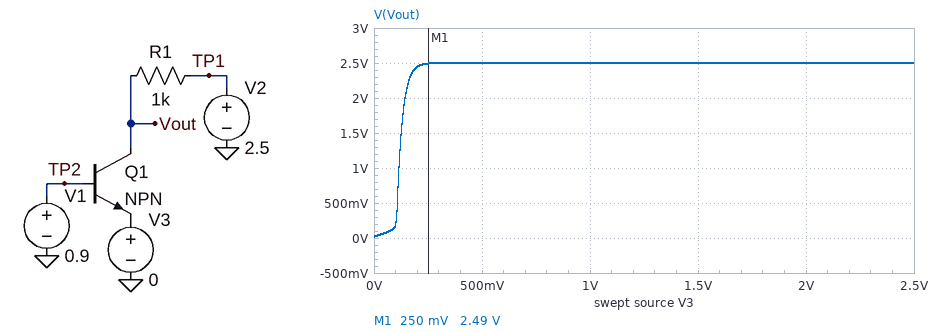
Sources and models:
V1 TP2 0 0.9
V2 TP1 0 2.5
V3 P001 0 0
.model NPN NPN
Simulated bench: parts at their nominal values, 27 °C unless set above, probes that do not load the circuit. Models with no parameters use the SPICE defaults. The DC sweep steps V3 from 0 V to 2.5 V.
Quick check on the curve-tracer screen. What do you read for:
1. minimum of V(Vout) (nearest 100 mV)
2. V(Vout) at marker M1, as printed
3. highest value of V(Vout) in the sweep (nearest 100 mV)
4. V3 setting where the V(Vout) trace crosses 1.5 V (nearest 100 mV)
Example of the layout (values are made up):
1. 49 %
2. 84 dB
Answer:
1. 0 V
2. 2.49 V
3. 2.5 V
4. 100 mV
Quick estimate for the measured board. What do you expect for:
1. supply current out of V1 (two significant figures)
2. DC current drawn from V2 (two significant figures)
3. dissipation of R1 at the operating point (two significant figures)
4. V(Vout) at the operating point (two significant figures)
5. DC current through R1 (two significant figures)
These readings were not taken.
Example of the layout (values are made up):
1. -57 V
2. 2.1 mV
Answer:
1. 65 mA
2. 2.5 mA
3. 6.2 mW
4. 18 mV
5. 2.5 mA
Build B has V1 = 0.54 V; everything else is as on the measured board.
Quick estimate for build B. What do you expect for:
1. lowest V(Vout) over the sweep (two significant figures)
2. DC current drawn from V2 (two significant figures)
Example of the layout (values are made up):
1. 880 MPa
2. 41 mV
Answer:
1. 2.5 V
2. 120 nA
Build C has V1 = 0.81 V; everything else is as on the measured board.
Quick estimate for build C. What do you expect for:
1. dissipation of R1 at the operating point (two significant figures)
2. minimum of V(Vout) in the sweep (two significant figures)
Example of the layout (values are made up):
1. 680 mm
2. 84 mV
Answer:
1. 6.0 mW
2. 43 mV
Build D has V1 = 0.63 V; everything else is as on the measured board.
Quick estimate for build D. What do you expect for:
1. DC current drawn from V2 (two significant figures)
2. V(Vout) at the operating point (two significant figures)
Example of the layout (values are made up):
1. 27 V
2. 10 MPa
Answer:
1. 3.8 µA
2. 2.5 V
